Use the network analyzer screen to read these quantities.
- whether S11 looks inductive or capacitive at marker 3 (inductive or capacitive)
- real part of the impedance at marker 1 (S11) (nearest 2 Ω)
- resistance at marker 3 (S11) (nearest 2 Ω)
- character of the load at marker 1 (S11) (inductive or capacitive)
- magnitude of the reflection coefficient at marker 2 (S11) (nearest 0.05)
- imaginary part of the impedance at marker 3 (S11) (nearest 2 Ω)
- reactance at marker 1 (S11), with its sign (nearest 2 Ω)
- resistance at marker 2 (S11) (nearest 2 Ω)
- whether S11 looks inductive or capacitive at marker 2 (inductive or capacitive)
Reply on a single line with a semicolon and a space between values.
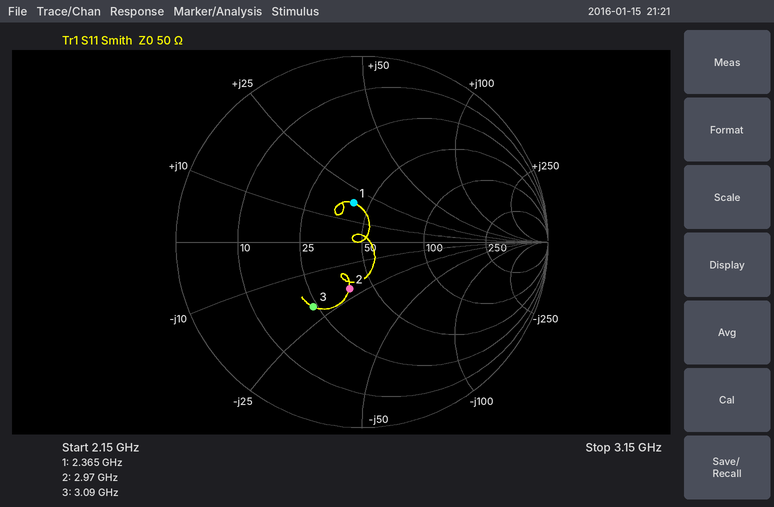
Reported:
capacitive; 42 Ω; 24 Ω; inductive; 0.25; -20 Ω; +18 Ω; 38 Ω; capacitive
